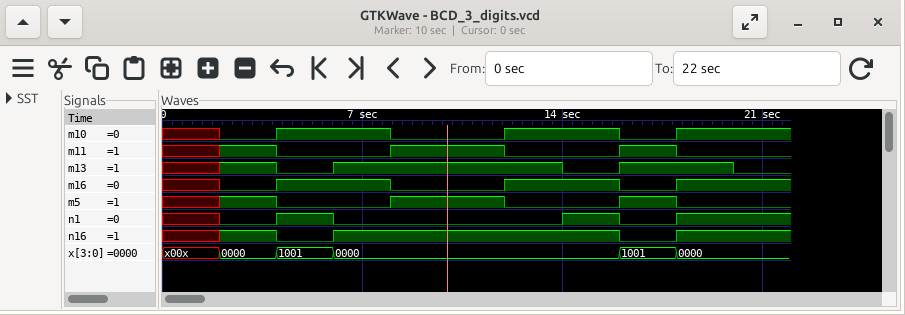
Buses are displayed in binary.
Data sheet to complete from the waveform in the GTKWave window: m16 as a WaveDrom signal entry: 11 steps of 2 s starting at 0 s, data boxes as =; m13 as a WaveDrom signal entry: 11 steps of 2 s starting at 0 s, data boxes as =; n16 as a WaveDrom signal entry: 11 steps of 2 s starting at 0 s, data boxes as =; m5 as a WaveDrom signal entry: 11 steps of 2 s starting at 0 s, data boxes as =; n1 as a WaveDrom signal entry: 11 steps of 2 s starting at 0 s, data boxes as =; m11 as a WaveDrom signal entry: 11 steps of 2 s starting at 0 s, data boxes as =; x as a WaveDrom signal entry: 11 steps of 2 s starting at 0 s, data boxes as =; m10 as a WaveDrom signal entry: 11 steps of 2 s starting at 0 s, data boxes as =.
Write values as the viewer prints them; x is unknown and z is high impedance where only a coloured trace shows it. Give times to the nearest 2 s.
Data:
{name: 'm16', wave: 'x01.0.1.01.'}
{name: 'm13', wave: 'x101...01.0'}
{name: 'n16', wave: 'x101....01.'}
{name: 'm5', wave: 'x10.1.0.10.'}
{name: 'n1', wave: 'x010...101.'}
{name: 'm11', wave: 'x10.1.0.10.'}
{name: 'x', wave: '====....==.', data: 'x00x 0000 1001 0000 1001 0000'}
{name: 'm10', wave: 'x01.0.1.01.'}
